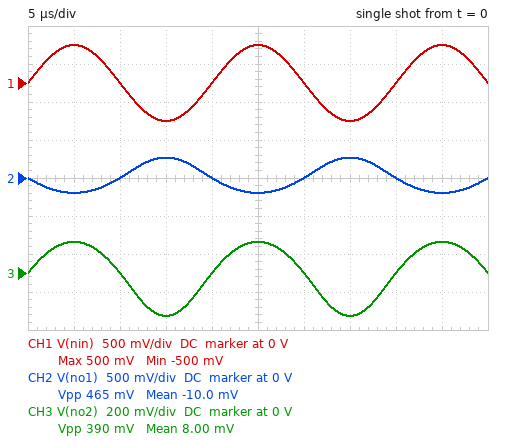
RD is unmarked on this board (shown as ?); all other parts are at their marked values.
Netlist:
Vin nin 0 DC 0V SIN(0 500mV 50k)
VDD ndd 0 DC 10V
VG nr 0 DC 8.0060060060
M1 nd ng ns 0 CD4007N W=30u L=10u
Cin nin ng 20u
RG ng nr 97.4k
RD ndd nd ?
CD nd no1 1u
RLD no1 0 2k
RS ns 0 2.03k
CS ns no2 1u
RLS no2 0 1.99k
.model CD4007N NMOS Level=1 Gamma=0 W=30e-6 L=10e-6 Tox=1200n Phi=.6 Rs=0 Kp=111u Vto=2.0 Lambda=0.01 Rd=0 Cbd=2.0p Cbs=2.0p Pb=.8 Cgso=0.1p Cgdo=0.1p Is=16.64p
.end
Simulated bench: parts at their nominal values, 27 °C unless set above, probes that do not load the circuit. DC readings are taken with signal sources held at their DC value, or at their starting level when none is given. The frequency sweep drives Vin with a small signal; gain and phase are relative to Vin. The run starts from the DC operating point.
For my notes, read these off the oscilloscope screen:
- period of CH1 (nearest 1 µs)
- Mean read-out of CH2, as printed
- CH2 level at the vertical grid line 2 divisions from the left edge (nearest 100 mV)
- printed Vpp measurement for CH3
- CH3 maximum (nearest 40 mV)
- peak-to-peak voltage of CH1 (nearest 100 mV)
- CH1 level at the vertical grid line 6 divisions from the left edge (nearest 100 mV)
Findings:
20 µs
-10.0 mV
0 V
390 mV
160 mV
1.0 V
0 V
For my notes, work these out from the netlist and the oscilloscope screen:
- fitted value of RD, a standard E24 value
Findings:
3 kΩ
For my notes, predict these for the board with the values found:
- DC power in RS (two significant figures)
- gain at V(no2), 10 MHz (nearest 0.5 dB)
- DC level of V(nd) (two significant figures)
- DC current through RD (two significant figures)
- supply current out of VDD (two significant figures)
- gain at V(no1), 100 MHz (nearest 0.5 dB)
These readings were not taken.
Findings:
4.5 mW
-8.5 dB
5.5 V
1.5 mA
1.5 mA
-7.0 dB
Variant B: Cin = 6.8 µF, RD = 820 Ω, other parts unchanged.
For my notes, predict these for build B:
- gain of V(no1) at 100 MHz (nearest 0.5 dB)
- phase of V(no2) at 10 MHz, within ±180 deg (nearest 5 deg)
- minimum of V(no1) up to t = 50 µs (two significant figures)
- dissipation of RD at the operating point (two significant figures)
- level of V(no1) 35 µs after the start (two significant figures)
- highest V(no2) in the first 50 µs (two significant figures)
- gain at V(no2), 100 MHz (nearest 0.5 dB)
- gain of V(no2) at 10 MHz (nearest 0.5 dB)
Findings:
-10.0 dB
0 deg
-150 mV
1.9 mW
140 mV
260 mV
-6.5 dB
-6.0 dB
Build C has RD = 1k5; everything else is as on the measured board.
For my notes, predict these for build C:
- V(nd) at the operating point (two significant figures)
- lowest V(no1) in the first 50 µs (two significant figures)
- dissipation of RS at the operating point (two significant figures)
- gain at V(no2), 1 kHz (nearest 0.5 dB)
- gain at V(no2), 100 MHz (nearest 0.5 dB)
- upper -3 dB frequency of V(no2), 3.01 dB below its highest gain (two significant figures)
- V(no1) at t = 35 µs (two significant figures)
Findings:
7.7 V
-220 mV
4.6 mW
-6.0 dB
-6.5 dB
350 MHz
210 mV
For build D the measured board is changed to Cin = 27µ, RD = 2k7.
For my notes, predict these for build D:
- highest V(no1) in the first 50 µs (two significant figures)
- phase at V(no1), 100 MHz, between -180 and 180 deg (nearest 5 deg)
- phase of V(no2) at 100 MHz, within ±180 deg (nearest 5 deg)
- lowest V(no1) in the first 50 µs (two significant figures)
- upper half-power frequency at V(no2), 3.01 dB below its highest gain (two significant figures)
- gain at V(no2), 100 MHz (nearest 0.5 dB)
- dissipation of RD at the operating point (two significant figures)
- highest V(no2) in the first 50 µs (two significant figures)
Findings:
280 mV
170 deg
-15 deg
-230 mV
360 MHz
-6.5 dB
6.1 mW
200 mV
